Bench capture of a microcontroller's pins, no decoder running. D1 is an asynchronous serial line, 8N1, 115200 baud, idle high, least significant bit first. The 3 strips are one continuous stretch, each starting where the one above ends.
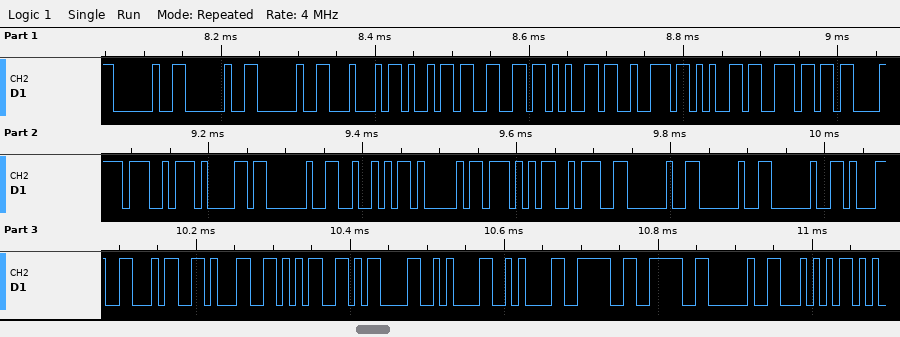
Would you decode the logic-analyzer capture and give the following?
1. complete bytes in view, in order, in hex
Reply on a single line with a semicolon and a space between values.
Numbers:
20 20 20 44 69 66 65 72 65 6E C3 A7 61 20 52 41 57 3A 20 20 20 31 34 31 35 0D 0A 0A 3E 3E 20 54
